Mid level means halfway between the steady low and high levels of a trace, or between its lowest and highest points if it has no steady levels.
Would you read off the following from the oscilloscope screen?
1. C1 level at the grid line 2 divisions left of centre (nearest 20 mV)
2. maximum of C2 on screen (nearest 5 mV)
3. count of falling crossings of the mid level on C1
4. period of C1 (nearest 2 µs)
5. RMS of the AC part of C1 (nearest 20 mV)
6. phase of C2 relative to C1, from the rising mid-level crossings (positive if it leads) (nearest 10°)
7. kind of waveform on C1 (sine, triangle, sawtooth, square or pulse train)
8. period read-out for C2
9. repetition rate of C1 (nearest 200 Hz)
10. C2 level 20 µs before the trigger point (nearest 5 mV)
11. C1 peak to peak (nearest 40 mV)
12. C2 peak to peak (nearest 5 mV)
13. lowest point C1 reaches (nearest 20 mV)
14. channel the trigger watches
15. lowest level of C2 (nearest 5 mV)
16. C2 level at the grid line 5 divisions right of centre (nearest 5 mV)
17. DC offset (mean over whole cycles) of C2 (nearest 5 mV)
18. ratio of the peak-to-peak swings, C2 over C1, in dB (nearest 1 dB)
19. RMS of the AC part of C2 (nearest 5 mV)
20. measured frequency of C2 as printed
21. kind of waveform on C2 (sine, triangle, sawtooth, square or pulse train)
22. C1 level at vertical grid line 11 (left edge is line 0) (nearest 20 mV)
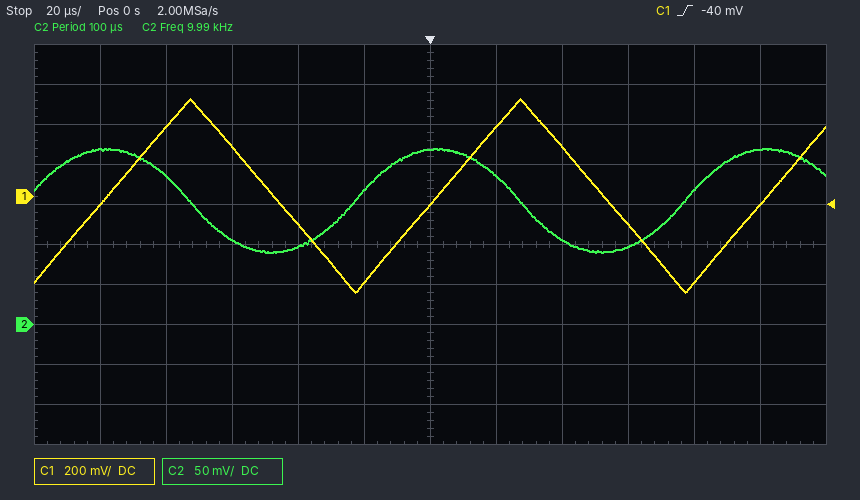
-140 mV
220 mV
2
100 µs
280 mV
+90°
triangle
100 µs
10.0 kHz
170 mV
960 mV
130 mV
-480 mV
C1
90 mV
220 mV
155 mV
-17 dB
45 mV
9.99 kHz
sine
-40 mV
